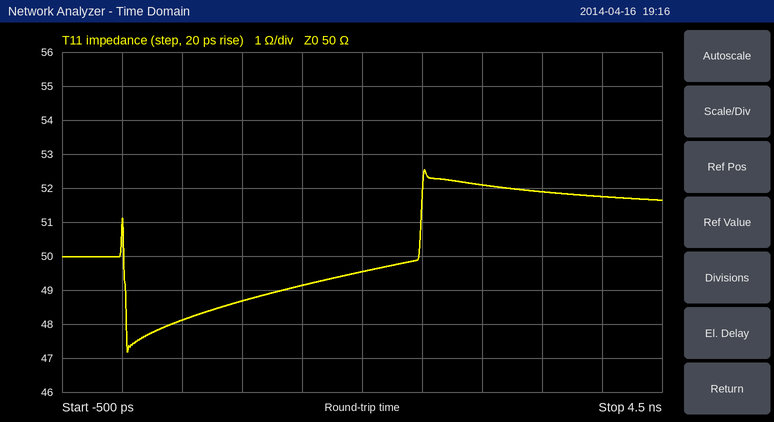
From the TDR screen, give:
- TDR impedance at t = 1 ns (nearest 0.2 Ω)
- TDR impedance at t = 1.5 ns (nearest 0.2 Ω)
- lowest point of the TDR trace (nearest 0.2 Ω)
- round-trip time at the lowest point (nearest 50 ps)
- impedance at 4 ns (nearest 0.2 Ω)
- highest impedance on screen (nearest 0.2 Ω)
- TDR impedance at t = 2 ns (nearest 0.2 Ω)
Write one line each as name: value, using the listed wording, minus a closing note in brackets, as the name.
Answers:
TDR impedance at t = 1 ns: 48.6 Ω
TDR impedance at t = 1.5 ns: 49.2 Ω
lowest point of the TDR trace: 47.2 Ω
round-trip time at the lowest point: 50 ps
impedance at 4 ns: 51.8 Ω
highest impedance on screen: 52.6 Ω
TDR impedance at t = 2 ns: 49.6 Ω
